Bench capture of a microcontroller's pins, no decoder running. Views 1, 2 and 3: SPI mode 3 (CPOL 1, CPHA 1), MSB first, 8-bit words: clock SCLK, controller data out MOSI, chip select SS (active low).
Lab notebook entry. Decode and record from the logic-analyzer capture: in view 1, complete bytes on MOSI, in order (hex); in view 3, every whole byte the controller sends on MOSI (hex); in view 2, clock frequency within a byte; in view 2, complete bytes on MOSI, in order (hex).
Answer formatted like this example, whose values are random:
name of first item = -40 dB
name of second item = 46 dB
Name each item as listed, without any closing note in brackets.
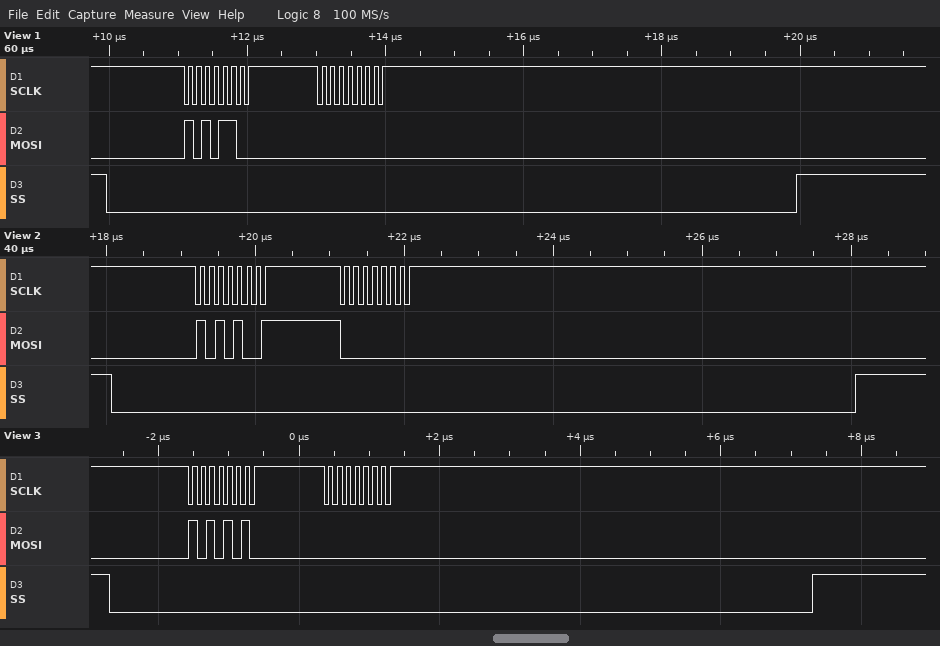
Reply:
in view 1, complete bytes on MOSI, in order = 0xAC 0x00
in view 3, every whole byte the controller sends on MOSI = AA 00
in view 2, clock frequency within a byte = 8 MHz
in view 2, complete bytes on MOSI, in order = A9 00
